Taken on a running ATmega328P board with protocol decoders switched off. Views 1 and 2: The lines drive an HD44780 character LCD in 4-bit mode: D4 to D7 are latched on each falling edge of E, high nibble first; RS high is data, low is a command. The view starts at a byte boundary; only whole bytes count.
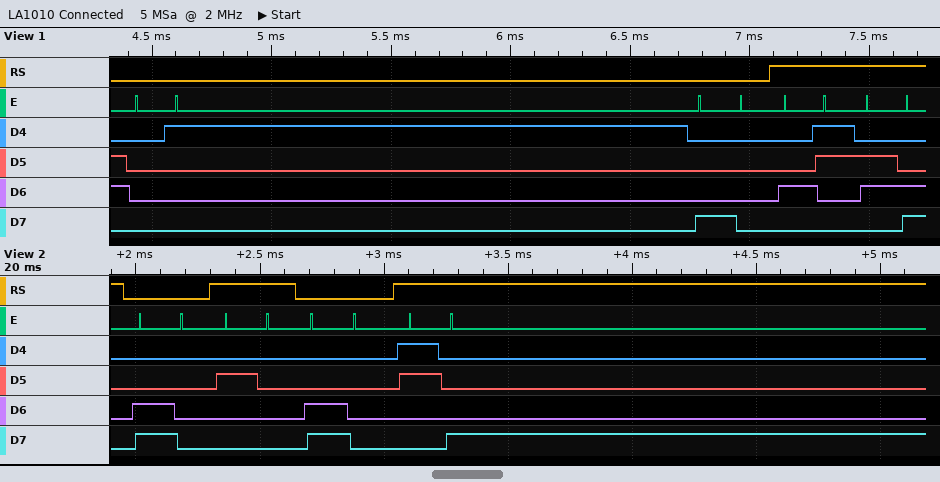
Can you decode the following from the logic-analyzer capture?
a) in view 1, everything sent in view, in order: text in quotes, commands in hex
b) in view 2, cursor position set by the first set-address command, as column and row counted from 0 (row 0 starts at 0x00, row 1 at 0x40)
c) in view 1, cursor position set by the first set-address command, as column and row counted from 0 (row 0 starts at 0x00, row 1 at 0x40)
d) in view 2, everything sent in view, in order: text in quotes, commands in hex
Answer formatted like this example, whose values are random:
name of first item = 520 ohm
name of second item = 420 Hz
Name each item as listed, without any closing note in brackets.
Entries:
in view 1, everything sent in view, in order: text in quotes, commands in hex = 0x01 0x80 "Cl"
in view 2, cursor position set by the first set-address command, as column and row counted from 0 = column 0, row 1
in view 1, cursor position set by the first set-address command, as column and row counted from 0 = column 0, row 0
in view 2, everything sent in view, in order: text in quotes, commands in hex = 0xC0 " " 0xC0 "8"
